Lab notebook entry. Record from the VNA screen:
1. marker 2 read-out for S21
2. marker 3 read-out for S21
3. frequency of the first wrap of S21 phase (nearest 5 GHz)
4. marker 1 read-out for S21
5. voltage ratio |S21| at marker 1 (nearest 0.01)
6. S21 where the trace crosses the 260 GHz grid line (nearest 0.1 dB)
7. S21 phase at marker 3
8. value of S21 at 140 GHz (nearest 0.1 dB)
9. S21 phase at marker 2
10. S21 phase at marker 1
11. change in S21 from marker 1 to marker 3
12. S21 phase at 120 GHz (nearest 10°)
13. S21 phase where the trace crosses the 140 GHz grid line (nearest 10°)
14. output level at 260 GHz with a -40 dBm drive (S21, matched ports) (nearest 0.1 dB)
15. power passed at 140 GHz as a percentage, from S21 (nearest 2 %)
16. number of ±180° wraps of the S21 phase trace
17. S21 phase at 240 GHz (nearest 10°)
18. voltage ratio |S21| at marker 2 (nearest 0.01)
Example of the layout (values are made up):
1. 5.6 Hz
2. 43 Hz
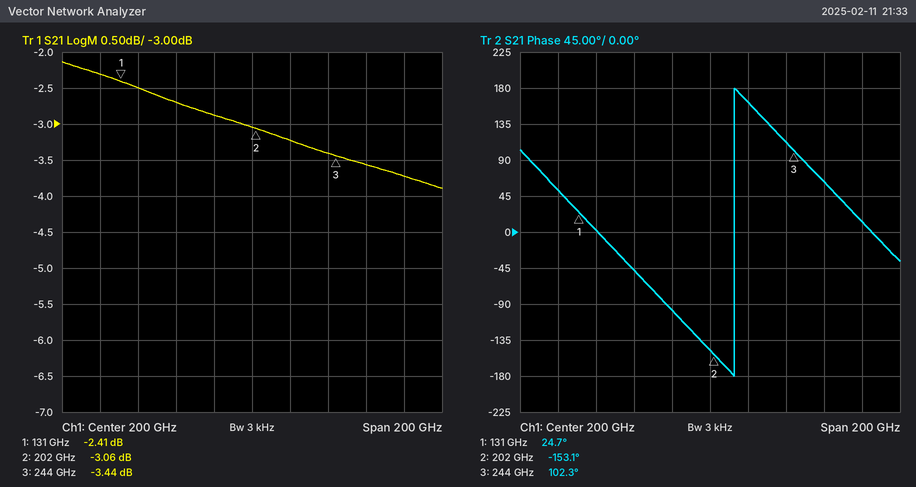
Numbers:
1. -3.06 dB
2. -3.44 dB
3. 215 GHz
4. -2.41 dB
5. 0.76
6. -3.6 dB
7. 102.3°
8. -2.5 dB
9. -153.1°
10. 24.7°
11. -1.03 dB
12. 50°
13. 0°
14. -43.6 dBm
15. 56 %
16. 1
17. 110°
18. 0.70
